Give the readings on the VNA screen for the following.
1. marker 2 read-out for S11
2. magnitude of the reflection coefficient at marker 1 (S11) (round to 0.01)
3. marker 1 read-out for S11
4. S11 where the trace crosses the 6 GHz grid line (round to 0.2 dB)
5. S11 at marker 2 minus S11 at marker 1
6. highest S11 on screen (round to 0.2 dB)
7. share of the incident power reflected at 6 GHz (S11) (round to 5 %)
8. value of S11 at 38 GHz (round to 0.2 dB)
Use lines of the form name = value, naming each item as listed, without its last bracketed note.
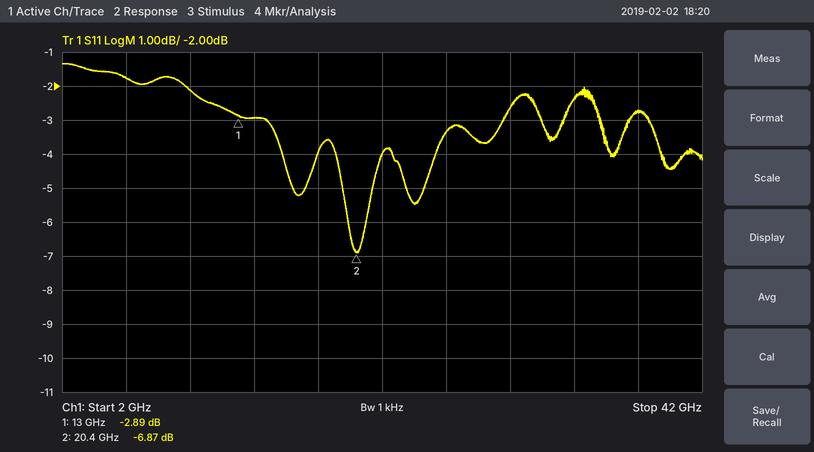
marker 2 read-out for S11 = -6.87 dB
magnitude of the reflection coefficient at marker 1 (S11) = 0.72
marker 1 read-out for S11 = -2.89 dB
S11 where the trace crosses the 6 GHz grid line = -1.8 dB
S11 at marker 2 minus S11 at marker 1 = -3.98 dB
highest S11 on screen = -1.4 dB
share of the incident power reflected at 6 GHz (S11) = 65 %
value of S11 at 38 GHz = -2.8 dB
